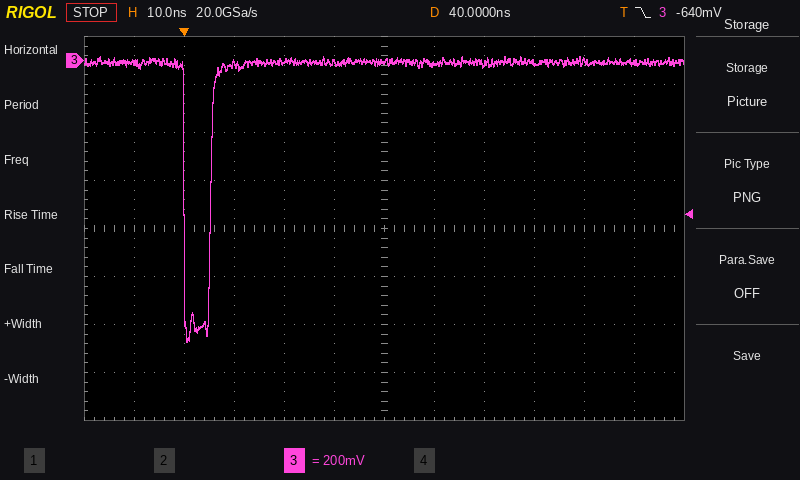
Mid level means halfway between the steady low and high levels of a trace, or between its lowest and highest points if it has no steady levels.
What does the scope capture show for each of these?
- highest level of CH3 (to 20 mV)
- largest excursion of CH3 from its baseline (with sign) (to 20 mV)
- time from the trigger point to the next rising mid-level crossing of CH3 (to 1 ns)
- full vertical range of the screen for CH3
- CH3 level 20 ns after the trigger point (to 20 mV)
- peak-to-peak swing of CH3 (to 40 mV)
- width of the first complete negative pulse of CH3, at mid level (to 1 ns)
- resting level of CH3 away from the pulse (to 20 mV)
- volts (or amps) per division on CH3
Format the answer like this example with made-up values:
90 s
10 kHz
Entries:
20 mV
-1.16 V
5 ns
1.6 V
0 mV
1.20 V
5 ns
0 mV
200 mV
